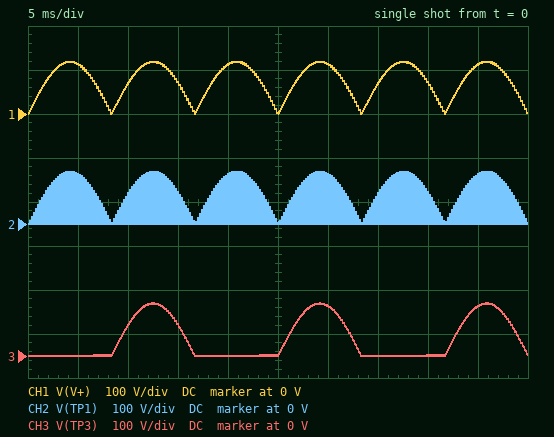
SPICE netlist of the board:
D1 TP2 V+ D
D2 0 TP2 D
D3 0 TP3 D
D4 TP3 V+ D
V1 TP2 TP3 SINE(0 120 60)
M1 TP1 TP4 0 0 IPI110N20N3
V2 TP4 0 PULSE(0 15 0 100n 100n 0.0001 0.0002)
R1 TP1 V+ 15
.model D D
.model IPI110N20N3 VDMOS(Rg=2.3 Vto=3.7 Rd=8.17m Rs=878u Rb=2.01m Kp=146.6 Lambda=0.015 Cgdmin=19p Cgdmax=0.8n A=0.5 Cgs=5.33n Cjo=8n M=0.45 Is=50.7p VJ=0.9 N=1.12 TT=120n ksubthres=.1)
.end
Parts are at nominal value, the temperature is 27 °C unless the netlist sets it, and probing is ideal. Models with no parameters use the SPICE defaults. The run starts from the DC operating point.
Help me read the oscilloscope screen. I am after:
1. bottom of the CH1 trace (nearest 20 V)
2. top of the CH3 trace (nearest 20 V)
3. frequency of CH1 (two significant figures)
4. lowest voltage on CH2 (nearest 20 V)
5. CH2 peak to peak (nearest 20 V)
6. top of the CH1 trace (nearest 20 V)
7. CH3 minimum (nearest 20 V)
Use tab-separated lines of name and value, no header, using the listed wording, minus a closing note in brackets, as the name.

bottom of the CH1 trace	0 V
top of the CH3 trace	120 V
frequency of CH1	120 Hz
lowest voltage on CH2	0 V
CH2 peak to peak	120 V
top of the CH1 trace	120 V
CH3 minimum	0 V
